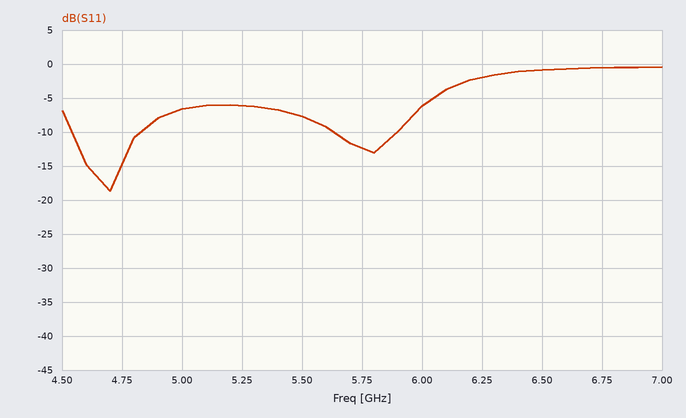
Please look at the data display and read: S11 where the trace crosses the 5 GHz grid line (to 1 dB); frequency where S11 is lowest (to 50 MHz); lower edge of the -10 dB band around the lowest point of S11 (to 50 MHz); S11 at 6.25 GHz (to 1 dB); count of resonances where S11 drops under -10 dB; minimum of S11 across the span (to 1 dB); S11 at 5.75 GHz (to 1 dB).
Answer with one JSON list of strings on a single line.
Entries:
["-7 dB", "4.70 GHz", "4.55 GHz", "-2 dB", "2", "-19 dB", "-12 dB"]
